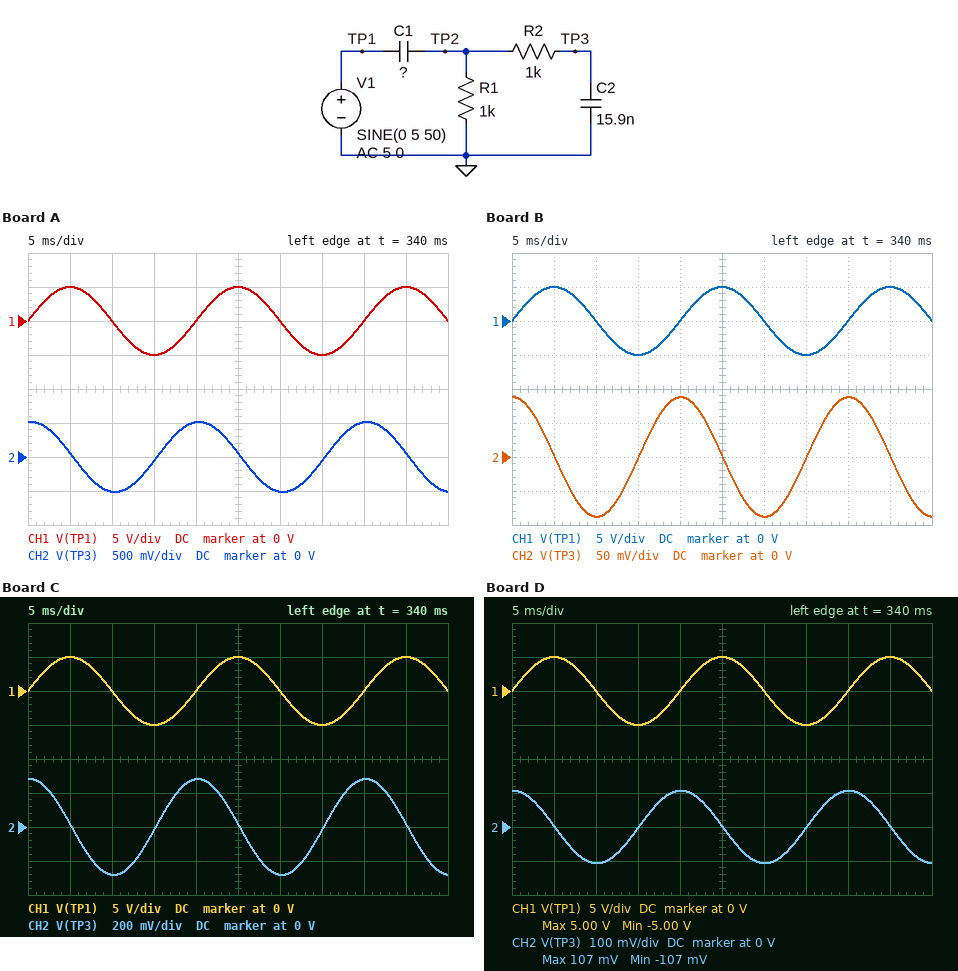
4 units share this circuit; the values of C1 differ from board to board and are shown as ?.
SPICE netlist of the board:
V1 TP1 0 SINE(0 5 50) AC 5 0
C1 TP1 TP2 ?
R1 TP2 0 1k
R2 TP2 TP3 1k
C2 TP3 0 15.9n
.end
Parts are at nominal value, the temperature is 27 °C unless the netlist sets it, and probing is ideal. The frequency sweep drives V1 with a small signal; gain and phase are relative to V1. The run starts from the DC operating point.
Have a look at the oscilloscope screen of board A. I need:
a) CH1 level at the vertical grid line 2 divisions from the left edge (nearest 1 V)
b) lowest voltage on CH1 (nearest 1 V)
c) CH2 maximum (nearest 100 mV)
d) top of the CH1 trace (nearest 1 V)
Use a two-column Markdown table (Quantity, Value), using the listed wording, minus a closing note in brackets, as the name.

| Quantity | Value |
|---|---|
| CH1 level at the vertical grid line 2 divisions from the left edge | 0 V |
| lowest voltage on CH1 | -5 V |
| CH2 maximum | 500 mV |
| top of the CH1 trace | 5 V |
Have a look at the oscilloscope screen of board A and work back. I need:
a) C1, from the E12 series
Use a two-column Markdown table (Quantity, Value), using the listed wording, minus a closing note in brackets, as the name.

| Quantity | Value |
|---|---|
| C1, from the E12 series | 330 nF |
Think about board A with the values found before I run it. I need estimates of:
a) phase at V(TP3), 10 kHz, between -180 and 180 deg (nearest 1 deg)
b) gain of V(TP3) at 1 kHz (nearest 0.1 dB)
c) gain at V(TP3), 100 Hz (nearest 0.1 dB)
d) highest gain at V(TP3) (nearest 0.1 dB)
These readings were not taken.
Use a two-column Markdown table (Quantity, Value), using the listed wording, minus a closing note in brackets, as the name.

| Quantity | Value |
|---|---|
| phase at V(TP3), 10 kHz, between -180 and 180 deg | -41 deg |
| gain of V(TP3) at 1 kHz | -1.3 dB |
| gain at V(TP3), 100 Hz | -13.9 dB |
| highest gain at V(TP3) | -0.8 dB |
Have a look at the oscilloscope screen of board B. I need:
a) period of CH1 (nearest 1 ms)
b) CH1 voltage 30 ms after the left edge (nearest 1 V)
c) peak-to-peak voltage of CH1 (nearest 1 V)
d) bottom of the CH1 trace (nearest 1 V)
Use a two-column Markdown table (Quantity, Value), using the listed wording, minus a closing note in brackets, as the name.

| Quantity | Value |
|---|---|
| period of CH1 | 20 ms |
| CH1 voltage 30 ms after the left edge | 0 V |
| peak-to-peak voltage of CH1 | 10 V |
| bottom of the CH1 trace | -5 V |
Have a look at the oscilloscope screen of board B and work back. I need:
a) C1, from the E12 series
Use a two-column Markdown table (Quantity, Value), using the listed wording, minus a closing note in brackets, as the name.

| Quantity | Value |
|---|---|
| C1, from the E12 series | 56 nF |
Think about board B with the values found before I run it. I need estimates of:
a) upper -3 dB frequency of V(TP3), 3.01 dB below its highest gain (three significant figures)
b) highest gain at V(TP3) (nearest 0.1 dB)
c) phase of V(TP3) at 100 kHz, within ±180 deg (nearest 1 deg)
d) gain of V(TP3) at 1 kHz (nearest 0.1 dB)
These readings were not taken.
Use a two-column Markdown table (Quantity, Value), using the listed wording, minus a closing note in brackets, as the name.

| Quantity | Value |
|---|---|
| upper -3 dB frequency of V(TP3), 3.01 dB below its highest gain | 17.3 kHz |
| highest gain at V(TP3) | -3.9 dB |
| phase of V(TP3) at 100 kHz, within ±180 deg | -81 deg |
| gain of V(TP3) at 1 kHz | -10.0 dB |
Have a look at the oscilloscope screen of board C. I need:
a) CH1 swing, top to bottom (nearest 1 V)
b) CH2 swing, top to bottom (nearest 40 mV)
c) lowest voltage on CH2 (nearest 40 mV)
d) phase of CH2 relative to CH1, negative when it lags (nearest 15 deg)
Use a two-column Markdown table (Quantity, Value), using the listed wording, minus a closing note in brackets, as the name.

| Quantity | Value |
|---|---|
| CH1 swing, top to bottom | 10 V |
| CH2 swing, top to bottom | 560 mV |
| lowest voltage on CH2 | -280 mV |
| phase of CH2 relative to CH1, negative when it lags | 90 deg |
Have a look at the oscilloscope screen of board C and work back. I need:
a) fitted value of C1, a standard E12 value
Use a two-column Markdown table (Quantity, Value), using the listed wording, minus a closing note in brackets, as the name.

| Quantity | Value |
|---|---|
| fitted value of C1, a standard E12 value | 180 nF |
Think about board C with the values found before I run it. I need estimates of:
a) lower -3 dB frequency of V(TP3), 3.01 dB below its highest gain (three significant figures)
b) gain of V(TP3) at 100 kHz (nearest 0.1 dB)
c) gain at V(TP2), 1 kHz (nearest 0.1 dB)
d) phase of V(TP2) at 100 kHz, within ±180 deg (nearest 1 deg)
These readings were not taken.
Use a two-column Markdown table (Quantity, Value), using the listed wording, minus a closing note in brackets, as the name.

| Quantity | Value |
|---|---|
| lower -3 dB frequency of V(TP3), 3.01 dB below its highest gain | 709 Hz |
| gain of V(TP3) at 100 kHz | -20.0 dB |
| gain at V(TP2), 1 kHz | -3.0 dB |
| phase of V(TP2) at 100 kHz, within ±180 deg | 1 deg |
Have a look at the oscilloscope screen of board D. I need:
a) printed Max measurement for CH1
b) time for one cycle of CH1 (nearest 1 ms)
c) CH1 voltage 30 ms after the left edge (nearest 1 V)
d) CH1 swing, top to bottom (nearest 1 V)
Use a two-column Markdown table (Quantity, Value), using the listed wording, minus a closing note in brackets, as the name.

| Quantity | Value |
|---|---|
| printed Max measurement for CH1 | 5.00 V |
| time for one cycle of CH1 | 20 ms |
| CH1 voltage 30 ms after the left edge | 0 V |
| CH1 swing, top to bottom | 10 V |
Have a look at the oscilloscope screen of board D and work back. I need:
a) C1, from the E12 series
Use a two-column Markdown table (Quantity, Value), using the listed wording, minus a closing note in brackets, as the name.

| Quantity | Value |
|---|---|
| C1, from the E12 series | 68 nF |
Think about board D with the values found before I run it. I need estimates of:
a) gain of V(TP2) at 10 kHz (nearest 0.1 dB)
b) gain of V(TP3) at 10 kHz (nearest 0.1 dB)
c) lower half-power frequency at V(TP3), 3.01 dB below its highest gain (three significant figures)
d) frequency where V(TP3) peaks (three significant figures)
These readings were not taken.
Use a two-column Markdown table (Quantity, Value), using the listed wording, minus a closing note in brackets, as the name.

| Quantity | Value |
|---|---|
| gain of V(TP2) at 10 kHz | -1.4 dB |
| gain of V(TP3) at 10 kHz | -4.4 dB |
| lower half-power frequency at V(TP3), 3.01 dB below its highest gain | 1.45 kHz |
| frequency where V(TP3) peaks | 4.84 kHz |
